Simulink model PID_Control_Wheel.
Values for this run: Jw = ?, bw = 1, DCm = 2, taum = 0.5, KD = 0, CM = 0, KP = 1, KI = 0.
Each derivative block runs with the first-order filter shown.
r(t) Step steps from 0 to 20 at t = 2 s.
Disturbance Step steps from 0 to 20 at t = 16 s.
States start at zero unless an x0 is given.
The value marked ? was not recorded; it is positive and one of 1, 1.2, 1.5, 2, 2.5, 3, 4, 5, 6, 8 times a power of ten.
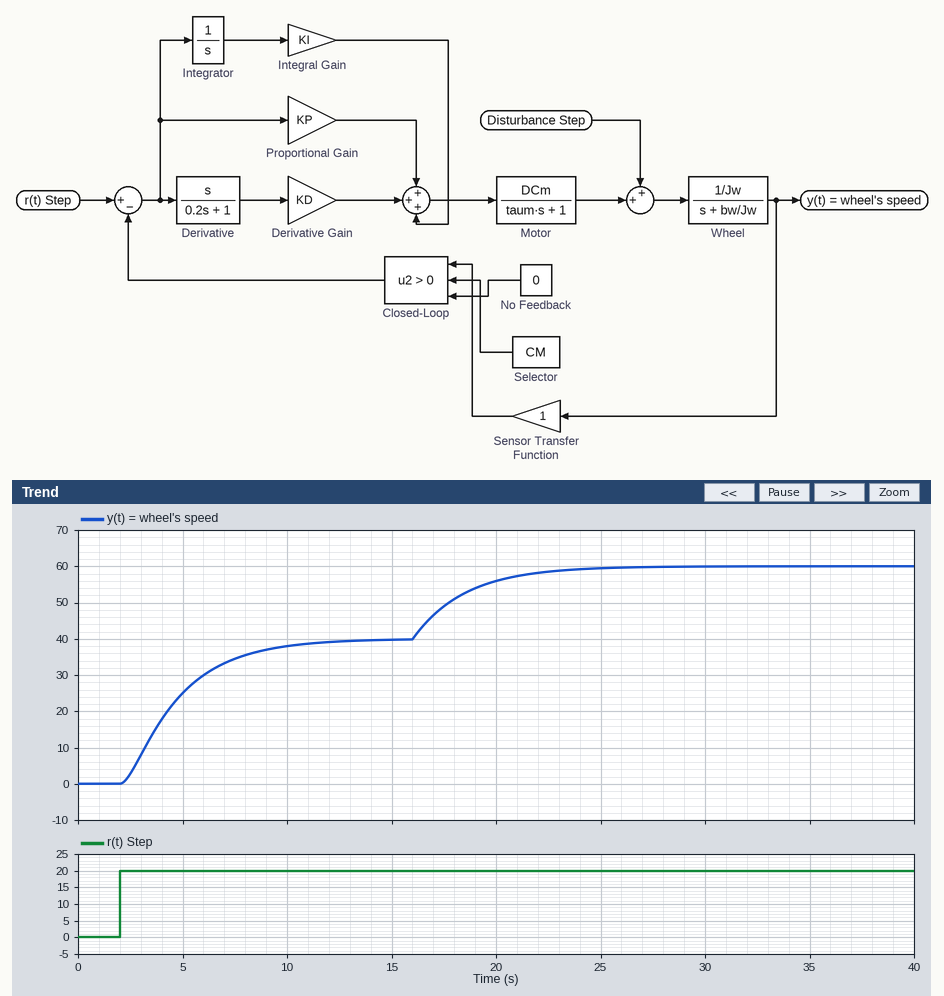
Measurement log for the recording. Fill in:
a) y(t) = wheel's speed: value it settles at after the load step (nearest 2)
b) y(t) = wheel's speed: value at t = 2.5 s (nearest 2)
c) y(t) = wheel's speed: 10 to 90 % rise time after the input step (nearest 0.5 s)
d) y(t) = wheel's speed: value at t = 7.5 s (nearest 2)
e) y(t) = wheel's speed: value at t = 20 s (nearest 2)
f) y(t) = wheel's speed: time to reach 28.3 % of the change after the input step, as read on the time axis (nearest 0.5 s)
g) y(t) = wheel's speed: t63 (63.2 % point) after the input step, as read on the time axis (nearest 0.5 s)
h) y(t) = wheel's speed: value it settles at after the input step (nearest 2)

60
2
5.5 s
34
56
3.5 s
5.0 s
40
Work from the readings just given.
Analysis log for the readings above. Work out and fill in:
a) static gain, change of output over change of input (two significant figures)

2.0
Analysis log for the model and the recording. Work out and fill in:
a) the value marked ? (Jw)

2.5
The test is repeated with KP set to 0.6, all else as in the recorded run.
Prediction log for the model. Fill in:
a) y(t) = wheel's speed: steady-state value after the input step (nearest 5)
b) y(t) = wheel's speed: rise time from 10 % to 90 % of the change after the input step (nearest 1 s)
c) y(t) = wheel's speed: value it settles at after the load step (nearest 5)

25
6 s
45
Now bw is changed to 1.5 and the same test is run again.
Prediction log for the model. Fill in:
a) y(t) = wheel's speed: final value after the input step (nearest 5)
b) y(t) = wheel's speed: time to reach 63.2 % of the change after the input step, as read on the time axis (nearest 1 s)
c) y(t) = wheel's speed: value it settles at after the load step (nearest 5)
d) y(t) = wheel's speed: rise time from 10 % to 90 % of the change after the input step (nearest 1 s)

25
4 s
40
4 s
